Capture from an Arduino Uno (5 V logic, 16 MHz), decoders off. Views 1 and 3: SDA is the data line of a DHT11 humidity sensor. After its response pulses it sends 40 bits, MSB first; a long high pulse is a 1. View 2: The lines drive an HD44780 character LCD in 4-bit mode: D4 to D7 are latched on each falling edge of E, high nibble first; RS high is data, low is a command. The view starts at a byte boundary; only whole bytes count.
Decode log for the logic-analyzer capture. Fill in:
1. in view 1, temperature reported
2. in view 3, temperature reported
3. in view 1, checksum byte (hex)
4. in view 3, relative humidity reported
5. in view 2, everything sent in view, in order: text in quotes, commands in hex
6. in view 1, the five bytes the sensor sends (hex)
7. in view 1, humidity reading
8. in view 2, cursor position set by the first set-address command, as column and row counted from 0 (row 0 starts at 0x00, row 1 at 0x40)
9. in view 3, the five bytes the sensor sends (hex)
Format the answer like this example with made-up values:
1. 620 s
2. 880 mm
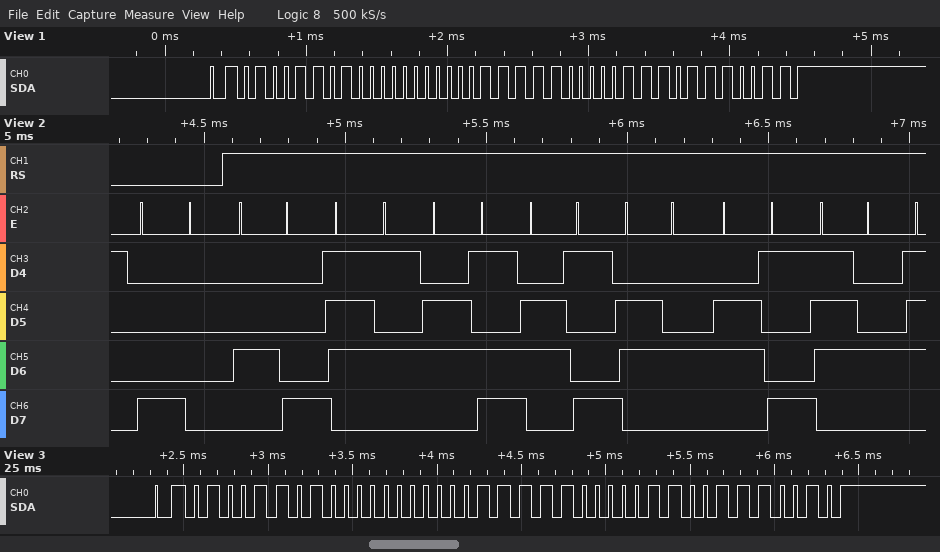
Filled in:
1. 31.7 °C
2. 31.6 °C
3. 0x73
4. 77 %
5. 0x80 "Humidit"
6. 4D 00 1F 07 73
7. 77 %
8. column 0, row 0
9. 4D 00 1F 06 72
